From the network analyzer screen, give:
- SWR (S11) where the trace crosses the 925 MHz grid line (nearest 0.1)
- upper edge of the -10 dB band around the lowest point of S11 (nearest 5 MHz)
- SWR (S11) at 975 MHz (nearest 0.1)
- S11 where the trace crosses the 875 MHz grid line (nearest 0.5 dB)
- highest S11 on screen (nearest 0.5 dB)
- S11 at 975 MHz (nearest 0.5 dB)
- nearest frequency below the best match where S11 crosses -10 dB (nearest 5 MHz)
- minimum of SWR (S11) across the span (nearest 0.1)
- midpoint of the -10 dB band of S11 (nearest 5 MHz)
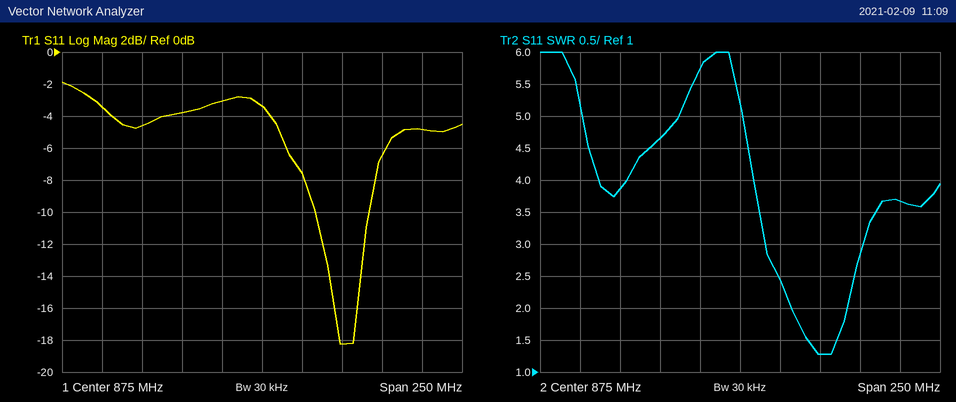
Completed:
1.3
940 MHz
3.7
-3.5 dB
-2.0 dB
-5.0 dB
910 MHz
1.3
925 MHz
